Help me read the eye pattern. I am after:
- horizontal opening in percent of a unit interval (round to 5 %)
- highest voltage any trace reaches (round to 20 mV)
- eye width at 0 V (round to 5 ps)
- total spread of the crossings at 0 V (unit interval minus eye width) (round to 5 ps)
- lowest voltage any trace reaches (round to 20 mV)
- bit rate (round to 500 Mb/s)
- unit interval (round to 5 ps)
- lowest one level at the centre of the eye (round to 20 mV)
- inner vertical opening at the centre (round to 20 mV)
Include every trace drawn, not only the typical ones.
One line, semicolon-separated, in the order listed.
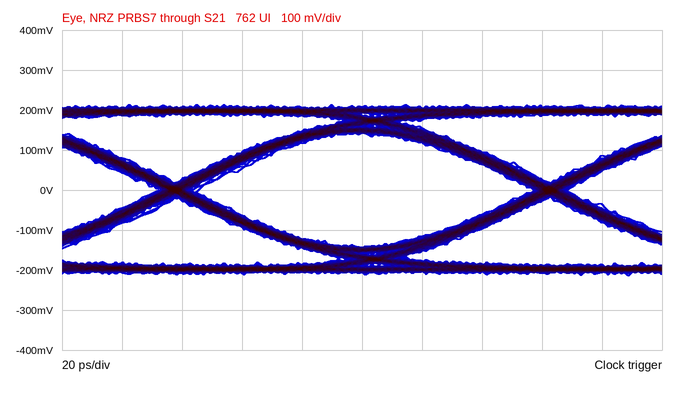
90 %; 220 mV; 110 ps; 15 ps; -220 mV; 8.0 Gb/s; 125 ps; 140 mV; 280 mV
